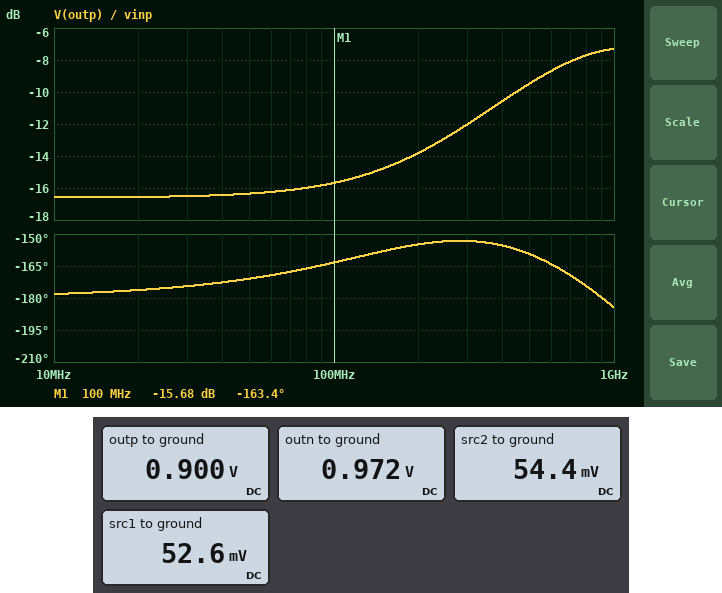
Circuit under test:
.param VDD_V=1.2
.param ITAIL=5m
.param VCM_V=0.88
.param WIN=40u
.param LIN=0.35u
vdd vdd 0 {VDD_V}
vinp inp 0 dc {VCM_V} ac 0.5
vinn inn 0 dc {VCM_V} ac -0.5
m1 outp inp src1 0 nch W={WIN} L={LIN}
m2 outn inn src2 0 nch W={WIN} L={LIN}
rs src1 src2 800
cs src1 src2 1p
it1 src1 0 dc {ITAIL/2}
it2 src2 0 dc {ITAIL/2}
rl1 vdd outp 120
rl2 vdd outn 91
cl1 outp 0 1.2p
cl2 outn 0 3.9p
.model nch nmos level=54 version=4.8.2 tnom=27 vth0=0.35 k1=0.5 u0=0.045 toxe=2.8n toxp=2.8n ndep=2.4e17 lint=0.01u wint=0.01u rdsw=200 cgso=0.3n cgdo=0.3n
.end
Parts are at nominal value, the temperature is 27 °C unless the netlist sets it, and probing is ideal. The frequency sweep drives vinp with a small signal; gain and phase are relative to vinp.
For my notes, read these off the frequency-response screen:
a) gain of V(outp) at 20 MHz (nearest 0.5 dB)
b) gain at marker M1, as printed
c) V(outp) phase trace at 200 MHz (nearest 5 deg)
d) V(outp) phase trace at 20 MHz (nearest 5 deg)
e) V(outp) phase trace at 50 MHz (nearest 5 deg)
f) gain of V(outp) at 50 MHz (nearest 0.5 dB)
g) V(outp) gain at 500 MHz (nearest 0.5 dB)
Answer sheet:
-16.5 dB
-15.68 dB
-155 deg
-175 deg
-170 deg
-16.5 dB
-9.5 dB
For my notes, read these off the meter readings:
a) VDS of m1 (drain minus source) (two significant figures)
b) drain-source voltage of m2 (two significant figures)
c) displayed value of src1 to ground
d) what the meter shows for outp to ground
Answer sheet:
850 mV
920 mV
52.6 mV
0.900 V
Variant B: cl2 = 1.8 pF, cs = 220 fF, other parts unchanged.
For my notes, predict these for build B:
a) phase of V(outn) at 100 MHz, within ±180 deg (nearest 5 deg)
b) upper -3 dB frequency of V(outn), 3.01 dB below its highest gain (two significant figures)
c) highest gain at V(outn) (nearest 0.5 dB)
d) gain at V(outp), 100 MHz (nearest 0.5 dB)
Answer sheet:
0 deg
5.3 GHz
-19.0 dB
-16.5 dB
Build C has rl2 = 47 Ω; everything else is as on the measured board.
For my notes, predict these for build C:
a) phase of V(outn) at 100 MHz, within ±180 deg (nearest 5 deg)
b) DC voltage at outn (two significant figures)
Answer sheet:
15 deg
1.1 V
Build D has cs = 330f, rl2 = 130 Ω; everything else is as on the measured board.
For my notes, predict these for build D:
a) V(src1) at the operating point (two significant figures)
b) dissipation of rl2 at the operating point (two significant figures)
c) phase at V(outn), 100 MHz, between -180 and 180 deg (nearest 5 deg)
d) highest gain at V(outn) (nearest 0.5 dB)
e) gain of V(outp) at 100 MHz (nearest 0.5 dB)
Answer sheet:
52 mV
810 µW
-10 deg
-16.0 dB
-16.5 dB
